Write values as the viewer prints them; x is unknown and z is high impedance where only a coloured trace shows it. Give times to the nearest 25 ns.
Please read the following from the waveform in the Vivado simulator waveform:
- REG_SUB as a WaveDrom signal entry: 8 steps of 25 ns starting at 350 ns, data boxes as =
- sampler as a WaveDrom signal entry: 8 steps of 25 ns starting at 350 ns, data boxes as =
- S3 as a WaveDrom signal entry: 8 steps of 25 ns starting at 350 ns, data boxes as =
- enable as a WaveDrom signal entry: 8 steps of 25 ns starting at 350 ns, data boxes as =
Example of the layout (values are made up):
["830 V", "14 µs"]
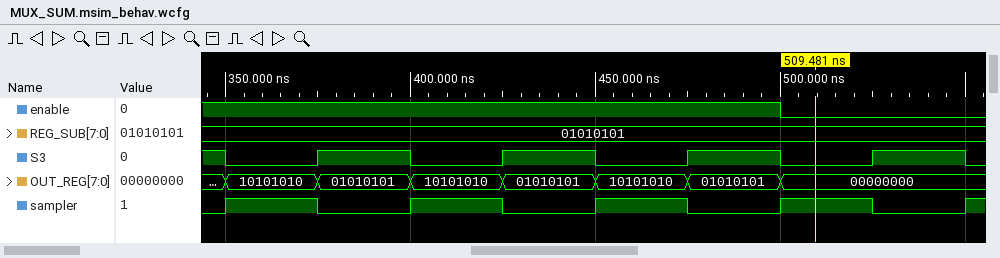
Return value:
["{name: 'REG_SUB', wave: '=.......', data: '01010101'}", "{name: 'sampler', wave: '10101010'}", "{name: 'S3', wave: '01010101'}", "{name: 'enable', wave: '1.....0.'}"]
